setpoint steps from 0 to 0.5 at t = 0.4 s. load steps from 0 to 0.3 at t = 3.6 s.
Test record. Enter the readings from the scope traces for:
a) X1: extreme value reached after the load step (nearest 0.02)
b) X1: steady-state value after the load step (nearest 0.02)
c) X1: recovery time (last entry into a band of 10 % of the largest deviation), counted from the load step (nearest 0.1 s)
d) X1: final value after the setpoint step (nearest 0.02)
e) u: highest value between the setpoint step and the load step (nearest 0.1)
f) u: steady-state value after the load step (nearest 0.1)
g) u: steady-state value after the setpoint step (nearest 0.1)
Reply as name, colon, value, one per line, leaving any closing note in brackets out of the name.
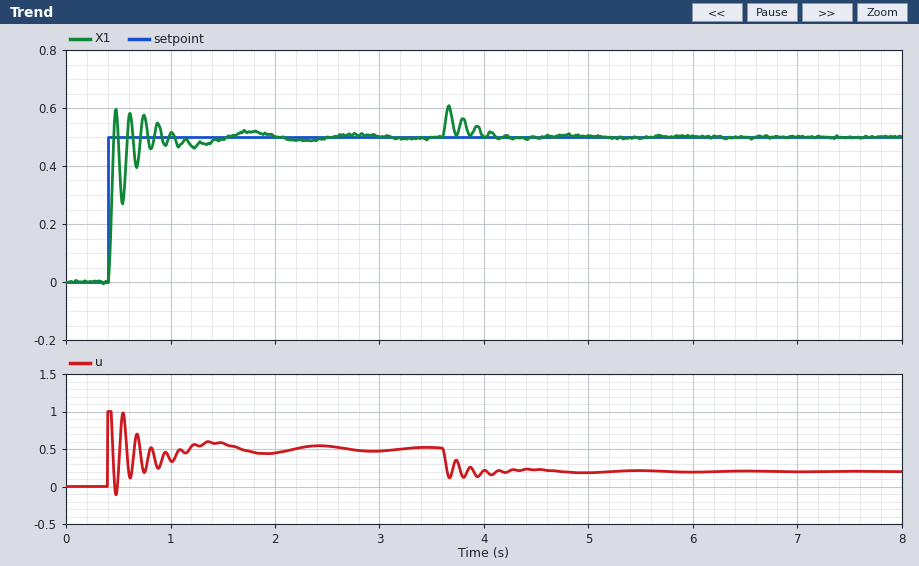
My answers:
X1: extreme value reached after the load step: 0.60
X1: steady-state value after the load step: 0.50
X1: recovery time (last entry into a band of 10 % of the largest deviation), counted from the load step: 0.5 s
X1: final value after the setpoint step: 0.50
u: highest value between the setpoint step and the load step: 1.0
u: steady-state value after the load step: 0.2
u: steady-state value after the setpoint step: 0.5
